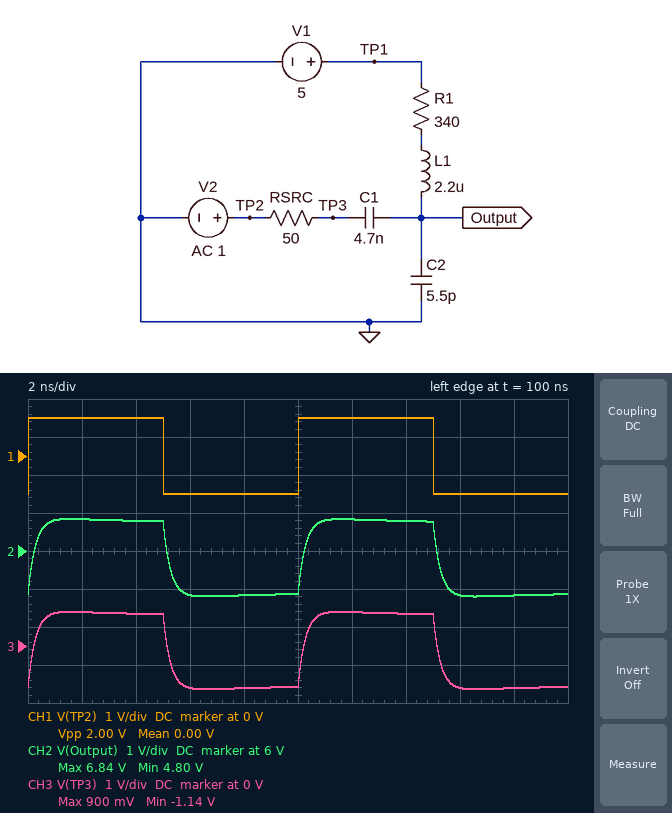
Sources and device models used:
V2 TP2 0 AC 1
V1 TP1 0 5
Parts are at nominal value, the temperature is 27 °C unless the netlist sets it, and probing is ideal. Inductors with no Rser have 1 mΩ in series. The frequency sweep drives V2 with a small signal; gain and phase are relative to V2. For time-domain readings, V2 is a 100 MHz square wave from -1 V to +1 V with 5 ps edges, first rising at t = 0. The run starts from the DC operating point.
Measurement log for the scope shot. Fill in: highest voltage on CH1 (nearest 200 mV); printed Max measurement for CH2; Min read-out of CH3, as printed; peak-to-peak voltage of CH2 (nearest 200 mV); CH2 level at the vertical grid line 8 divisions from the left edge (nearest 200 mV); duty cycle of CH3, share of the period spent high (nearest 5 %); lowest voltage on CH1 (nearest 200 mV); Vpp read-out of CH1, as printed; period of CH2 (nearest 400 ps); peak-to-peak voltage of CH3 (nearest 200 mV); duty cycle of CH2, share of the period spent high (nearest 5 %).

1.0 V
6.84 V
-1.14 V
2.0 V
4.8 V
50 %
-1.0 V
2.00 V
10.0 ns
2.0 V
50 %
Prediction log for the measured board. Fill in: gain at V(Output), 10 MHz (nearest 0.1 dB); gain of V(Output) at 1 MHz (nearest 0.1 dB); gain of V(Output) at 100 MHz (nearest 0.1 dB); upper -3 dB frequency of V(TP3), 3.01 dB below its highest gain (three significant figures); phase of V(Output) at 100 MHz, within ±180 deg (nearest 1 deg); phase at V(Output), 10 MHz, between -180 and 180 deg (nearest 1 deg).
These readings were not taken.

-1.0 dB
-1.2 dB
-0.2 dB
583 MHz
-8 deg
2 deg
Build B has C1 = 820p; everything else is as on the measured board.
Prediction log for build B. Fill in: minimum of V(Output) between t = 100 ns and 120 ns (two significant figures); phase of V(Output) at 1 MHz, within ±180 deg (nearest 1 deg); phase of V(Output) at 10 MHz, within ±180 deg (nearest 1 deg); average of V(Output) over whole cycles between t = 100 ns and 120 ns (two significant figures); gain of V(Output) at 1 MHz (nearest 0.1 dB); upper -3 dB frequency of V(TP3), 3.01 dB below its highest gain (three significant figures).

4.6 V
27 deg
4 deg
5.6 V
-2.1 dB
586 MHz
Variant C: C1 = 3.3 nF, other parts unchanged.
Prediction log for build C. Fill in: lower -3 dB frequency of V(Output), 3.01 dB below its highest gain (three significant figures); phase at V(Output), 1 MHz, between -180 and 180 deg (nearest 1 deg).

162 kHz
7 deg
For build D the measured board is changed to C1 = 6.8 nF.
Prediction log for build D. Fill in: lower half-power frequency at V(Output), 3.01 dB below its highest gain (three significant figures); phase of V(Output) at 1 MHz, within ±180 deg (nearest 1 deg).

79.0 kHz
4 deg
